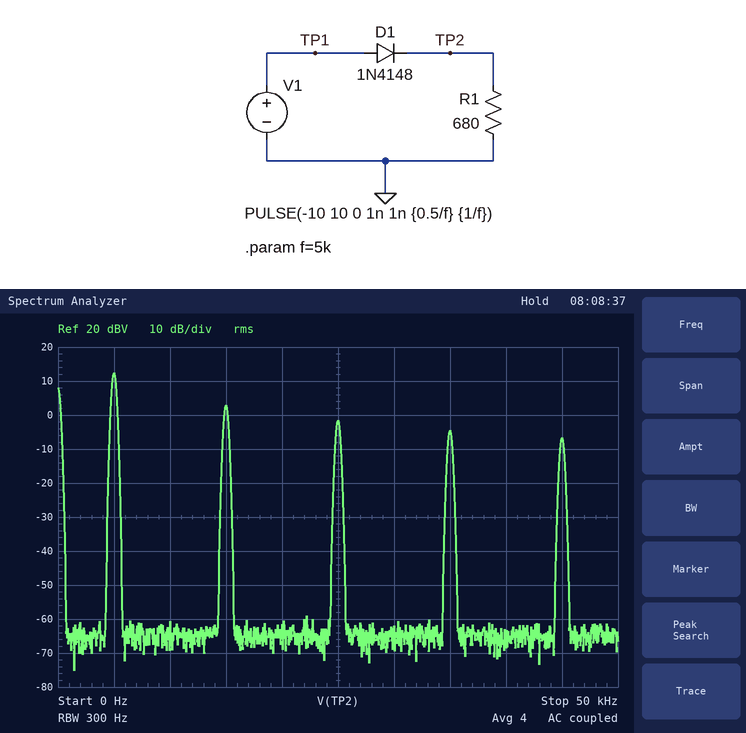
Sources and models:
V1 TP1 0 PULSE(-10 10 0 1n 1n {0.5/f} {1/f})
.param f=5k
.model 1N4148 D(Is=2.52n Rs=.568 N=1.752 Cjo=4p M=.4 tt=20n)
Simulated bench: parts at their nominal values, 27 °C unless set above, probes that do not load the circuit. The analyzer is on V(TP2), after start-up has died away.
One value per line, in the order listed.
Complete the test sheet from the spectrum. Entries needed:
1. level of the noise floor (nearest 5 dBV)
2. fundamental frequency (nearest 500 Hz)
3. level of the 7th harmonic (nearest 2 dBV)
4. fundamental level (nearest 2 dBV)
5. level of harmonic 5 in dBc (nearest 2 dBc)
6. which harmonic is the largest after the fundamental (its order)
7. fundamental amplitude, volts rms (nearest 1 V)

-65 dBV
5.0 kHz
-4 dBV
12 dBV
-14 dBc
3
4 V
